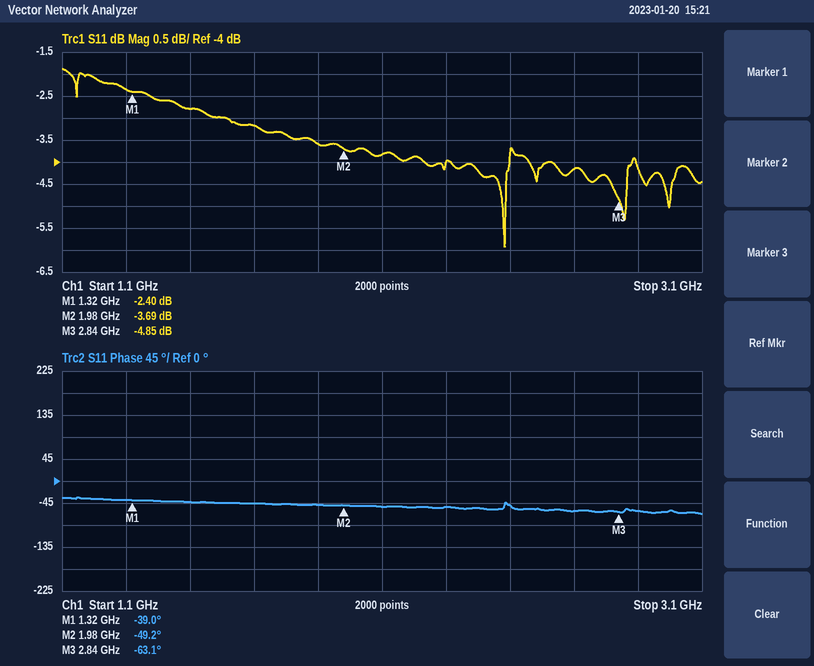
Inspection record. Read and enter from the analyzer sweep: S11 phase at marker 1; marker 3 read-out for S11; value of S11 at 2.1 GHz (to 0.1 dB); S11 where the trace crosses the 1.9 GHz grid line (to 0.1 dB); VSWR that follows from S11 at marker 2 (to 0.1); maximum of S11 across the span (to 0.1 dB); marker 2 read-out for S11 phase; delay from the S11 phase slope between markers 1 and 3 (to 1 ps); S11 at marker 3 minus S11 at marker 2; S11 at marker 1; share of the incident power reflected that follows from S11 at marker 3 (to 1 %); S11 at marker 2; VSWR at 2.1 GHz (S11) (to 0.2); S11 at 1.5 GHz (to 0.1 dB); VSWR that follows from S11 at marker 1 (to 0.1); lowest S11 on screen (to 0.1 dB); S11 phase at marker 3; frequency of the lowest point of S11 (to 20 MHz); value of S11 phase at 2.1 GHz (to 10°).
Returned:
-39.0°
-4.85 dB
-3.8 dB
-3.6 dB
4.8
-1.9 dB
-49.2°
44 ps
-1.16 dB
-2.40 dB
33 %
-3.69 dB
4.6
-2.8 dB
7.3
-5.9 dB
-63.1°
2.48 GHz
-50°
